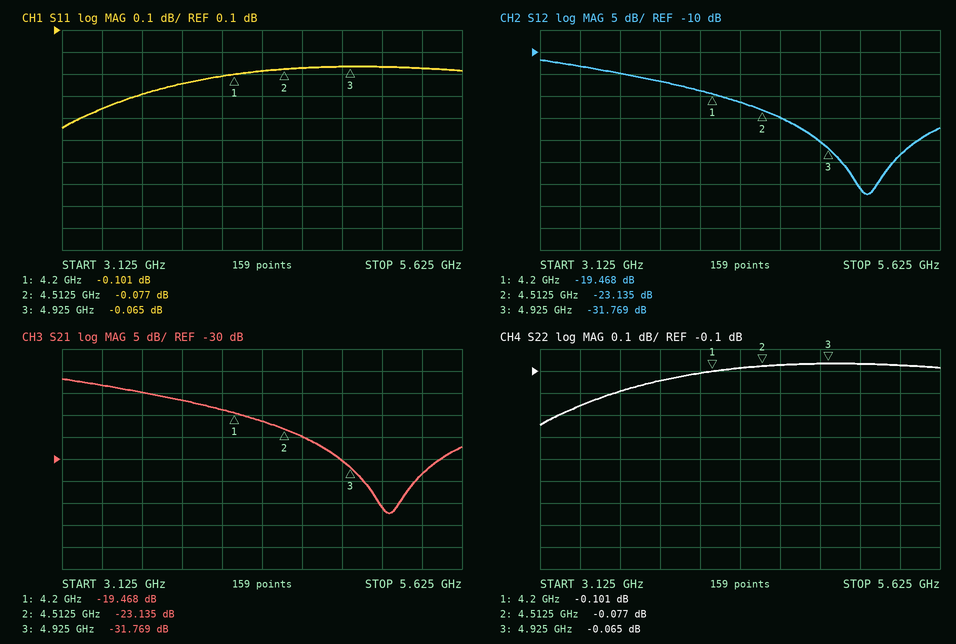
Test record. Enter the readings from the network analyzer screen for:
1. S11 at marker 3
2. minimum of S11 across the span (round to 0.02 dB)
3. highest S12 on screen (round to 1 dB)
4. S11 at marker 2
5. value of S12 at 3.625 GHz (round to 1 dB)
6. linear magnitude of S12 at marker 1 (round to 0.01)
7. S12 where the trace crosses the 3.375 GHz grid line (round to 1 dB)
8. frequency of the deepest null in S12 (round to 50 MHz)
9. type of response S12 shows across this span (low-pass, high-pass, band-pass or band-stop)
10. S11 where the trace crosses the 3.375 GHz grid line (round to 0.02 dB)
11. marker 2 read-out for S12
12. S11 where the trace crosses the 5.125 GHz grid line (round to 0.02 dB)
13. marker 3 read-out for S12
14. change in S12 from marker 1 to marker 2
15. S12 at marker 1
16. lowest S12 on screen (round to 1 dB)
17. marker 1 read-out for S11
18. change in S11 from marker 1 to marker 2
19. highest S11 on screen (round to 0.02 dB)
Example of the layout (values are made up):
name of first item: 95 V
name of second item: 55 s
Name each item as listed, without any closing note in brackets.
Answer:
S11 at marker 3: -0.065 dB
minimum of S11 across the span: -0.34 dB
highest S12 on screen: -12 dB
S11 at marker 2: -0.077 dB
value of S12 at 3.625 GHz: -15 dB
linear magnitude of S12 at marker 1: 0.11
S12 where the trace crosses the 3.375 GHz grid line: -13 dB
frequency of the deepest null in S12: 5.15 GHz
type of response S12 shows across this span: low-pass
S11 where the trace crosses the 3.375 GHz grid line: -0.26 dB
marker 2 read-out for S12: -23.135 dB
S11 where the trace crosses the 5.125 GHz grid line: -0.06 dB
marker 3 read-out for S12: -31.769 dB
change in S12 from marker 1 to marker 2: -3.667 dB
S12 at marker 1: -19.468 dB
lowest S12 on screen: -42 dB
marker 1 read-out for S11: -0.101 dB
change in S11 from marker 1 to marker 2: 0.024 dB
highest S11 on screen: -0.06 dB
